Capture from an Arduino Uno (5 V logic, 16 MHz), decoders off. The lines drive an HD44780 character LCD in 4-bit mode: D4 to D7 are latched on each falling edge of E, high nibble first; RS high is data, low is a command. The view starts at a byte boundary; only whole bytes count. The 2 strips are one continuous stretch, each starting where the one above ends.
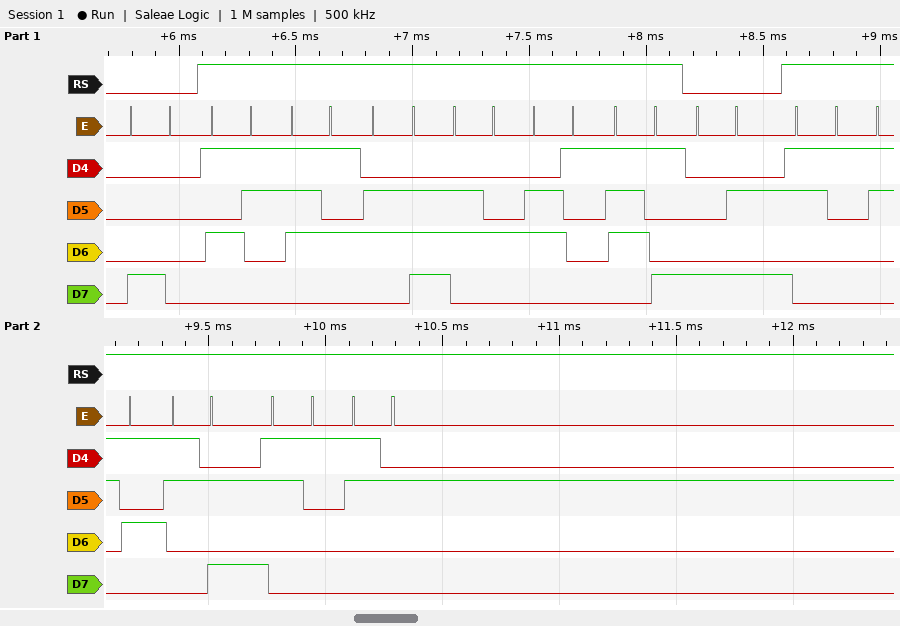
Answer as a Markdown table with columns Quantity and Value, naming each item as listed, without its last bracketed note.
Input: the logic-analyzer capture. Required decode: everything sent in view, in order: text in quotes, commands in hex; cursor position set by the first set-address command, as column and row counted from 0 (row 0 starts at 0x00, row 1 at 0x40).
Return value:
| Quantity | Value |
|---|---|
| everything sent in view, in order: text in quotes, commands in hex | 0x80 "Sunday" 0x8A "15:12" |
| cursor position set by the first set-address command, as column and row counted from 0 | column 0, row 0 |
